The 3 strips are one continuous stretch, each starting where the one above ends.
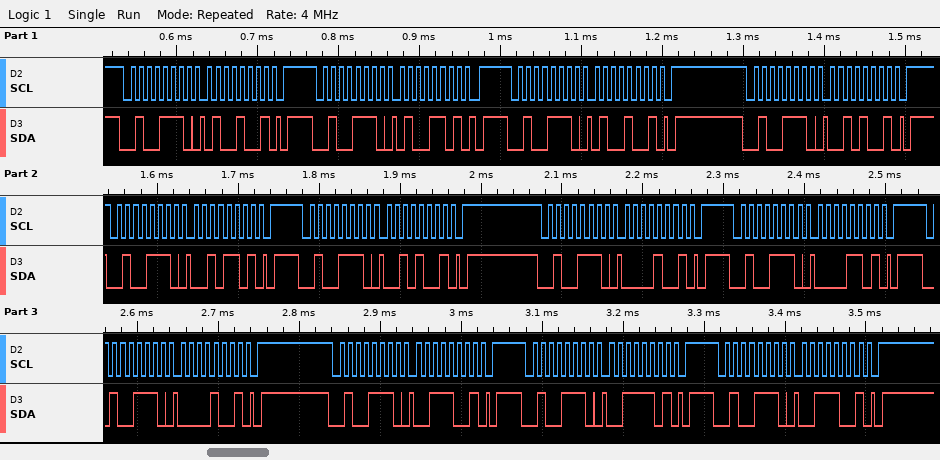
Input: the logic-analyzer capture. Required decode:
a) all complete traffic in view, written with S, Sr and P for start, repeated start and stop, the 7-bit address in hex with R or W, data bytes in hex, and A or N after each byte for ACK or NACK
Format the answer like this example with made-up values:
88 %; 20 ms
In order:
S 27W A 49 A P S 27W A 4D A P S 27W A 49 A P S 27W A 29 A P S 27W A 2D A P S 27W A 29 A P S 27W A 09 A P S 27W A 0D A P S 27W A 09 A P S 27W A 39 A P S 27W A 3D A P S 27W A 39 A P
